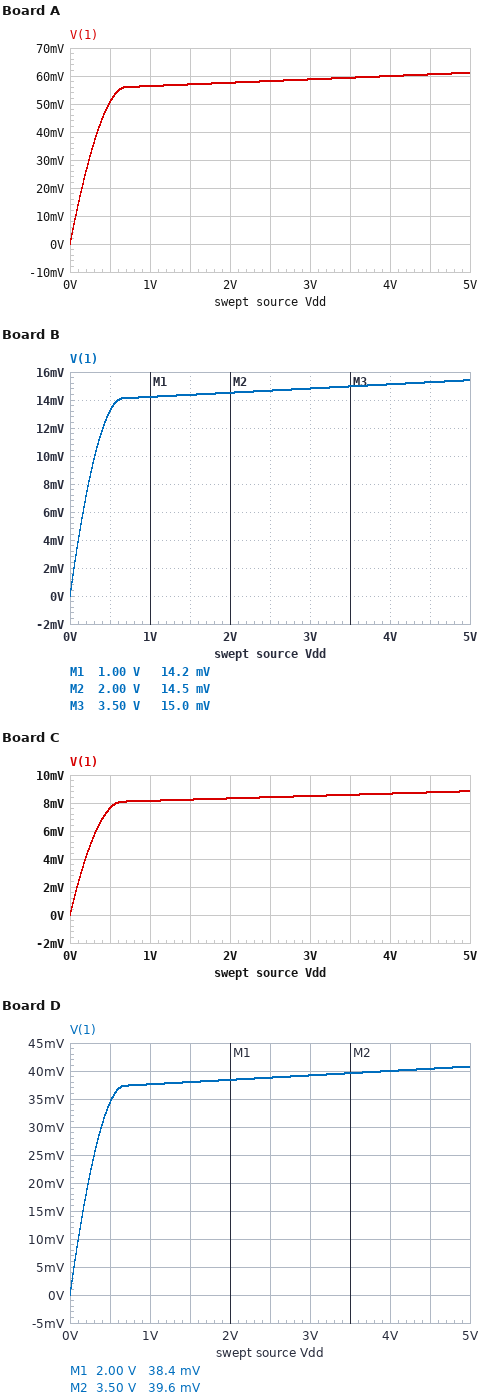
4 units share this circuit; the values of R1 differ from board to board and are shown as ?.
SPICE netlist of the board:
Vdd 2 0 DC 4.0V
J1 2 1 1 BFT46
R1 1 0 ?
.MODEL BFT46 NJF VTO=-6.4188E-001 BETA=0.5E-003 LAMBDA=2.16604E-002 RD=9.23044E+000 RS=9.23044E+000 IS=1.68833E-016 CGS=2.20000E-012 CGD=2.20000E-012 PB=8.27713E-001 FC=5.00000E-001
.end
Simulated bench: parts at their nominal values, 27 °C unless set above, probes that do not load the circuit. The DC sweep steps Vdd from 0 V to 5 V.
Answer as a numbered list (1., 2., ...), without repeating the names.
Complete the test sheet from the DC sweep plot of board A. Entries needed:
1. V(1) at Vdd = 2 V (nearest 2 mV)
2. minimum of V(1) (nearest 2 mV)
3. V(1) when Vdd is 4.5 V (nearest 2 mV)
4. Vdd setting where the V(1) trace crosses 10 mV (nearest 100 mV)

1. 58 mV
2. 0 V
3. 60 mV
4. 100 mV
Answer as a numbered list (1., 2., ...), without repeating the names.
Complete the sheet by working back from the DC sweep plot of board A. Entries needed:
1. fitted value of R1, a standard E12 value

1. 270 Ω
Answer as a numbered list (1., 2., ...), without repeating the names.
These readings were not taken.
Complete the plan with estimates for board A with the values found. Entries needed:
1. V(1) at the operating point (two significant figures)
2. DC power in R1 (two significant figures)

1. 60 mV
2. 13 µW
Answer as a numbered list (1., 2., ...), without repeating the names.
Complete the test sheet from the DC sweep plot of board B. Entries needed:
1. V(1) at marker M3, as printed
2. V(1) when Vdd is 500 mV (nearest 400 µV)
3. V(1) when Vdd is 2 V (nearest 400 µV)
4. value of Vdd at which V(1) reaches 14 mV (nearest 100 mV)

1. 15.0 mV
2. 13.2 mV
3. 14.4 mV
4. 600 mV
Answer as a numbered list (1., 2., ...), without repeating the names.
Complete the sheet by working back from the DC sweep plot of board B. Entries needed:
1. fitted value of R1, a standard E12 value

1. 68 Ω
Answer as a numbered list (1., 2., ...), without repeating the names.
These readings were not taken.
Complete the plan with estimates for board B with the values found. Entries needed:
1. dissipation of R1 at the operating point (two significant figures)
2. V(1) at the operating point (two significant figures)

1. 3.4 µW
2. 15 mV
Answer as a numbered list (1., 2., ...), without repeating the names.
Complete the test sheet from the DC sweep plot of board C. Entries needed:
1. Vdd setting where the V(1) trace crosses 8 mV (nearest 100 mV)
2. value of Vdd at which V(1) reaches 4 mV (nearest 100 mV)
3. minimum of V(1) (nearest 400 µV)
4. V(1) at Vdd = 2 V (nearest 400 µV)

1. 600 mV
2. 200 mV
3. 0 V
4. 8.4 mV
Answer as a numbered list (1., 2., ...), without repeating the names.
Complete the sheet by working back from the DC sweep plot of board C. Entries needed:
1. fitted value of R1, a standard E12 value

1. 39 Ω
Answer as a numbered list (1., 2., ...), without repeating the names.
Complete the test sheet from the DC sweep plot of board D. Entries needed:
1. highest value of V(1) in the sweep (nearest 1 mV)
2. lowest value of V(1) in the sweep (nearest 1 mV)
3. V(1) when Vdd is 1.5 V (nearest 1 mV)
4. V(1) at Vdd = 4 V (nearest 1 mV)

1. 41 mV
2. 0 V
3. 38 mV
4. 40 mV
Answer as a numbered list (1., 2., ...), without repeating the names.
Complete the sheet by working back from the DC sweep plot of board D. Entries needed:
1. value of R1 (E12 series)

1. 180 Ω
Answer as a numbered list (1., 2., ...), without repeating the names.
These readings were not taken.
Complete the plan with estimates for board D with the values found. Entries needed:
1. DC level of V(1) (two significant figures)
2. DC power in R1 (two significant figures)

1. 40 mV
2. 8.9 µW
